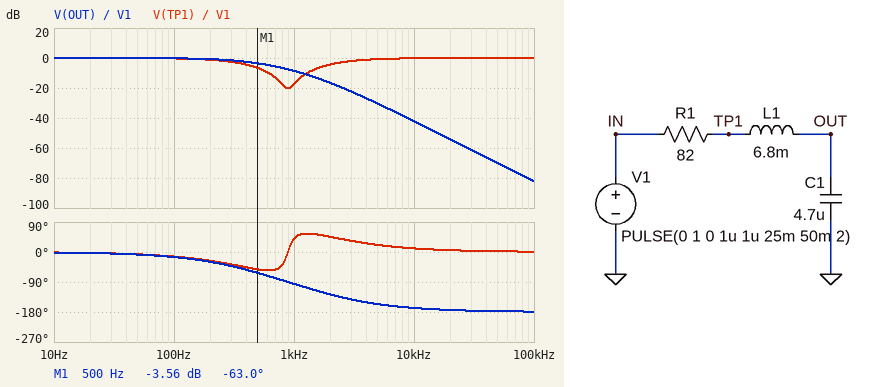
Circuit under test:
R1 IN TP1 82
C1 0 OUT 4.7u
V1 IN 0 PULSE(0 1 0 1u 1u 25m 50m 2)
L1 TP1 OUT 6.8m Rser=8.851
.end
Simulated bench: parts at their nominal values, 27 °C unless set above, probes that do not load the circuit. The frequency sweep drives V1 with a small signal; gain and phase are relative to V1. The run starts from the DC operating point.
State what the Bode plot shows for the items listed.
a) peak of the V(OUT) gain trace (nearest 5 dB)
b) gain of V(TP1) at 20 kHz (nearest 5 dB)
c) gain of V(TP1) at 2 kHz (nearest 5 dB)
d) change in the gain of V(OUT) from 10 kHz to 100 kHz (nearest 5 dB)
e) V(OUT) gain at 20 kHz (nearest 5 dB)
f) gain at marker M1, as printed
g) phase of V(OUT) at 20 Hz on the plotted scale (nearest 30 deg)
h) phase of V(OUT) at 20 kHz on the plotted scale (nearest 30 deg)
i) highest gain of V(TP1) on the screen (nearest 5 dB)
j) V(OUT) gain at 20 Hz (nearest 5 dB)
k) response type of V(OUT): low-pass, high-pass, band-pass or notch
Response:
0 dB
0 dB
-5 dB
-40 dB
-55 dB
-3.56 dB
0 deg
-180 deg
0 dB
0 dB
low-pass
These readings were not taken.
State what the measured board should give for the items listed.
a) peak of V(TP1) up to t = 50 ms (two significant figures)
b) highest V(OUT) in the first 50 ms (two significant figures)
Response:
1.0 V
1.0 V
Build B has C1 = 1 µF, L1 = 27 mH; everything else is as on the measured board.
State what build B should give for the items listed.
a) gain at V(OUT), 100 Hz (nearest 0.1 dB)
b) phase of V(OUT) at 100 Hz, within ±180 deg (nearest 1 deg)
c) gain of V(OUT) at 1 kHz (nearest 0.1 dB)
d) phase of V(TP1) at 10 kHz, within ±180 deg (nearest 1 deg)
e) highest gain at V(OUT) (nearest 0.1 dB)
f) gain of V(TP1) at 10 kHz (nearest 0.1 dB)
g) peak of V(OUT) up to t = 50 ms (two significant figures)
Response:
0.1 dB
-3 deg
4.8 dB
3 deg
5.5 dB
0 dB
1.4 V
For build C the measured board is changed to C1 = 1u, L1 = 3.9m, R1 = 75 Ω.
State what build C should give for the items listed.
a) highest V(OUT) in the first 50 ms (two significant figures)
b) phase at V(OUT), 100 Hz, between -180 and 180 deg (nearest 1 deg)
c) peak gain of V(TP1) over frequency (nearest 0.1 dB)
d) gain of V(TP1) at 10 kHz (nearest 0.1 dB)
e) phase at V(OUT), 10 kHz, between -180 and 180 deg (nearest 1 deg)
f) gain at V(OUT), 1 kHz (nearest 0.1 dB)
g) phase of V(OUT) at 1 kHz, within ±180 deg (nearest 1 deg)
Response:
1.1 V
-3 deg
0 dB
-0.5 dB
-160 deg
0 dB
-32 deg
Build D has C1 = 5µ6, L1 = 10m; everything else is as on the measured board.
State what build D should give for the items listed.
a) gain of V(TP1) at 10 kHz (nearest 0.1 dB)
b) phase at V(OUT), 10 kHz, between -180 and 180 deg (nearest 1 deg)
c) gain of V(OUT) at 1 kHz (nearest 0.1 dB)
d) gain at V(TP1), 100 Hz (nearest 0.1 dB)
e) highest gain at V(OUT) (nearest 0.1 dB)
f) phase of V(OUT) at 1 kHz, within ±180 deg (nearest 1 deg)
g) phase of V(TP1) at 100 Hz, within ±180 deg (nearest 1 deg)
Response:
-0.1 dB
-172 deg
-10.7 dB
-0.4 dB
0 dB
-111 deg
-16 deg
